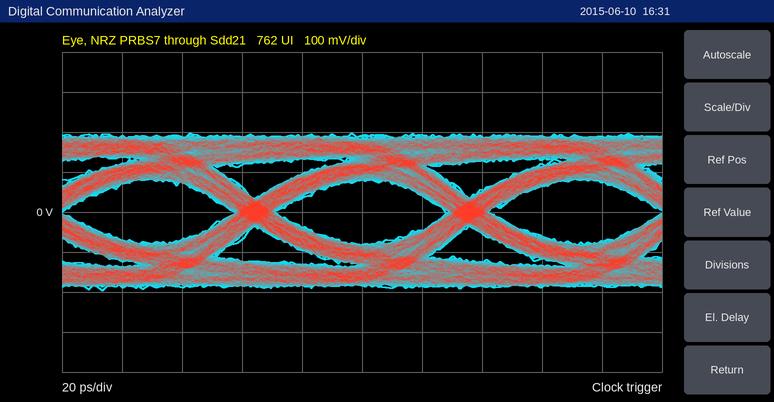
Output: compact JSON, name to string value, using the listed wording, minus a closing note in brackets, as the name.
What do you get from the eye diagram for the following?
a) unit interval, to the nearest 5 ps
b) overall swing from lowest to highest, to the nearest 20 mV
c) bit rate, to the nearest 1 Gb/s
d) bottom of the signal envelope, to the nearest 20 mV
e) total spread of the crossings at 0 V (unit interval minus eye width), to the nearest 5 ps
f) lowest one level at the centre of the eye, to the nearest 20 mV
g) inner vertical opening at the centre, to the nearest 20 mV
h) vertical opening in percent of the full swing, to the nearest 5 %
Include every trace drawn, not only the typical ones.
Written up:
{"unit interval, to the nearest 5 ps": "70 ps", "overall swing from lowest to highest, to the nearest 20 mV": "400 mV", "bit rate, to the nearest 1 Gb/s": "14 Gb/s", "bottom of the signal envelope, to the nearest 20 mV": "-200 mV", "total spread of the crossings at 0 V (unit interval minus eye width), to the nearest 5 ps": "15 ps", "lowest one level at the centre of the eye, to the nearest 20 mV": "80 mV", "inner vertical opening at the centre, to the nearest 20 mV": "160 mV", "vertical opening in percent of the full swing, to the nearest 5 %": "40 %"}
